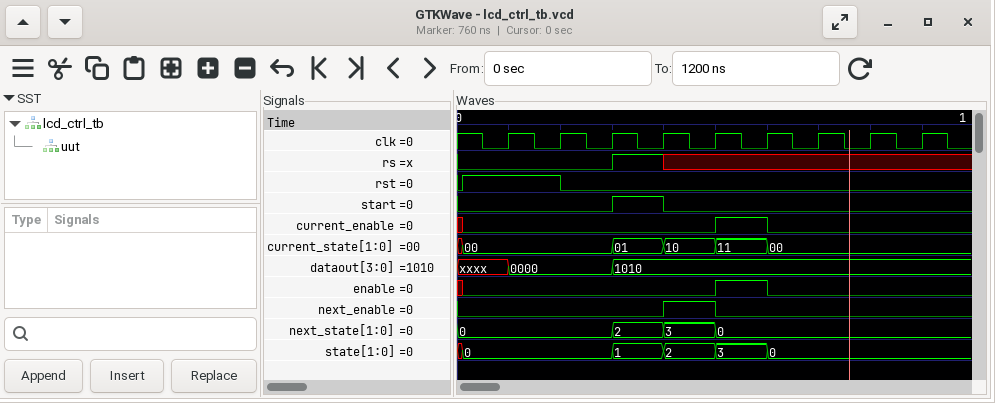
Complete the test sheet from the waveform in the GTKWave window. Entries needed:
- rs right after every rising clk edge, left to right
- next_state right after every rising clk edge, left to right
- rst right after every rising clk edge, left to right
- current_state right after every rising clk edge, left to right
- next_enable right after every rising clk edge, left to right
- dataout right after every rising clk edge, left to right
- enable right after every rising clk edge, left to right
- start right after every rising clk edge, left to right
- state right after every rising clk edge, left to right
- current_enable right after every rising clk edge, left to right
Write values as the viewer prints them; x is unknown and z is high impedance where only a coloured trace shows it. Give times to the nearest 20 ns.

0 0 1 x x x x x x
0, 0, 2, 3, 0, 0, 0, 0, 0
1 0 0 0 0 0 0 0 0
00, 00, 01, 10, 11, 00, 00, 00, 00
0 0 0 1 0 0 0 0 0
0000, 0000, 1010, 1010, 1010, 1010, 1010, 1010, 1010
0 0 0 0 1 0 0 0 0
0 0 1 0 0 0 0 0 0
0, 0, 1, 2, 3, 0, 0, 0, 0
0 0 0 0 1 0 0 0 0
